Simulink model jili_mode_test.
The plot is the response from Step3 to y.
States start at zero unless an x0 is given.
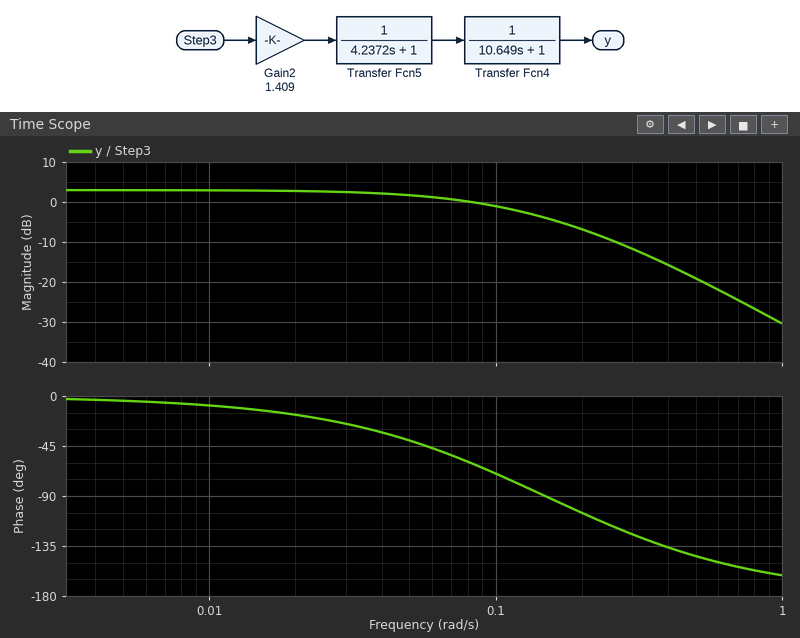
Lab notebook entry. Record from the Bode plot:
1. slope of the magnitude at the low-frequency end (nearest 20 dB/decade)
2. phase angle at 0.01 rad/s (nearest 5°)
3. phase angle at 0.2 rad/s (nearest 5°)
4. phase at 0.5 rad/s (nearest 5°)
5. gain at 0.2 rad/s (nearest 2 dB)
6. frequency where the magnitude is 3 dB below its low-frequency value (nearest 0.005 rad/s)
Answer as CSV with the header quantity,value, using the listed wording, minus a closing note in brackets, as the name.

quantity,value
slope of the magnitude at the low-frequency end,0 dB/decade
phase angle at 0.01 rad/s,-10°
phase angle at 0.2 rad/s,-105°
phase at 0.5 rad/s,-145°
gain at 0.2 rad/s,-6 dB
frequency where the magnitude is 3 dB below its low-frequency value,0.085 rad/s
